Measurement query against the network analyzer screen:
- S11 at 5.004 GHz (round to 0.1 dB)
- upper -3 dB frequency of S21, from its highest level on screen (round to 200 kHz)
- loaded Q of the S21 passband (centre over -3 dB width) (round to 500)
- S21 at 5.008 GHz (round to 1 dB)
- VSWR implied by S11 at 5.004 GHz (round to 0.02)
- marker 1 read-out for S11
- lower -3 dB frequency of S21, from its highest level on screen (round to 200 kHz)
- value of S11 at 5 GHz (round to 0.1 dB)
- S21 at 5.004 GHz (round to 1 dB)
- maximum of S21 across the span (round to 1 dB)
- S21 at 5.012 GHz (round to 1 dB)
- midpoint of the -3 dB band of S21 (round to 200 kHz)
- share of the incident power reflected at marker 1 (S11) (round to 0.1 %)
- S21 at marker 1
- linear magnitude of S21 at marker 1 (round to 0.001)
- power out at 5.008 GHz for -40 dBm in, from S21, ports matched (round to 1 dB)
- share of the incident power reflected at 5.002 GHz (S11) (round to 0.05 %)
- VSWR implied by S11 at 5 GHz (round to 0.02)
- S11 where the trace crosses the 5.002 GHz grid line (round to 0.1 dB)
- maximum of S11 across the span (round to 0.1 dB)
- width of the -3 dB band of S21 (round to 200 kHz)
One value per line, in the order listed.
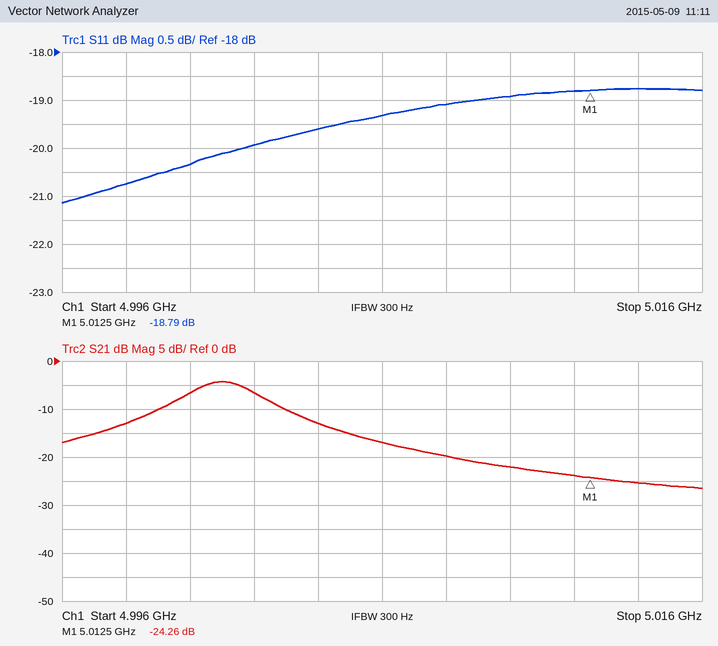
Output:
-19.6 dB
5.0022 GHz
2000
-20 dB
1.24
-18.79 dB
4.9998 GHz
-20.3 dB
-13 dB
-4 dB
-24 dB
5.0010 GHz
1.3 %
-24.26 dB
0.061
-60 dBm
1.00 %
1.22
-19.9 dB
-18.8 dB
2.4 MHz
